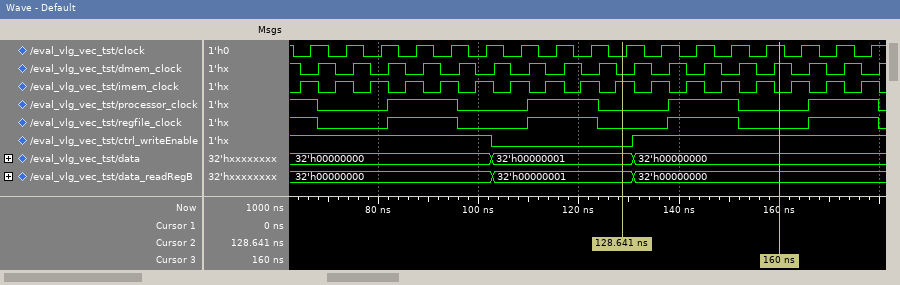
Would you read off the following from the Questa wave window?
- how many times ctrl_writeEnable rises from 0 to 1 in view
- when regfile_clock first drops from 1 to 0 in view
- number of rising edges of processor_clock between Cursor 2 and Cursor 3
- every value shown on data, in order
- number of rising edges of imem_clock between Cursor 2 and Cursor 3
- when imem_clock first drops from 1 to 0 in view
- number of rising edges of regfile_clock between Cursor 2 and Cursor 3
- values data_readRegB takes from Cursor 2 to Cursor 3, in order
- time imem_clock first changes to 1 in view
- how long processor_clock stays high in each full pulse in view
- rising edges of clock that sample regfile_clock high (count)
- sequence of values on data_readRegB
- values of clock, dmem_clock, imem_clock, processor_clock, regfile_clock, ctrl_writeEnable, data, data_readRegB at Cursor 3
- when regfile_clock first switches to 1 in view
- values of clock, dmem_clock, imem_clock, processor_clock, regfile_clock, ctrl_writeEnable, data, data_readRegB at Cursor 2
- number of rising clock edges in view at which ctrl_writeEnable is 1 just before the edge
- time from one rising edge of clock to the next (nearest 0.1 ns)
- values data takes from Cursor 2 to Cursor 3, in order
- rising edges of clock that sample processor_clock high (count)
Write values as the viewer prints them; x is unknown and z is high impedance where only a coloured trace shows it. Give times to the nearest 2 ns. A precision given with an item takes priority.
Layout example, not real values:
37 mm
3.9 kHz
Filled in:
1
68 ns
1
32'h00000000, 32'h00000001, 32'h00000000
4
68 ns
1
32'h00000001, 32'h00000000
64 ns
14 ns, 14 ns, 14 ns, 14 ns
9
32'h00000000, 32'h00000001, 32'h00000000
clock=1, dmem_clock=1, imem_clock=0, processor_clock=0, regfile_clock=0, ctrl_writeEnable=1, data=32'h00000000, data_readRegB=32'h00000000
82 ns
clock=0, dmem_clock=0, imem_clock=1, processor_clock=0, regfile_clock=0, ctrl_writeEnable=0, data=32'h00000001, data_readRegB=32'h00000001
13
7 ns
32'h00000001, 32'h00000000
9
